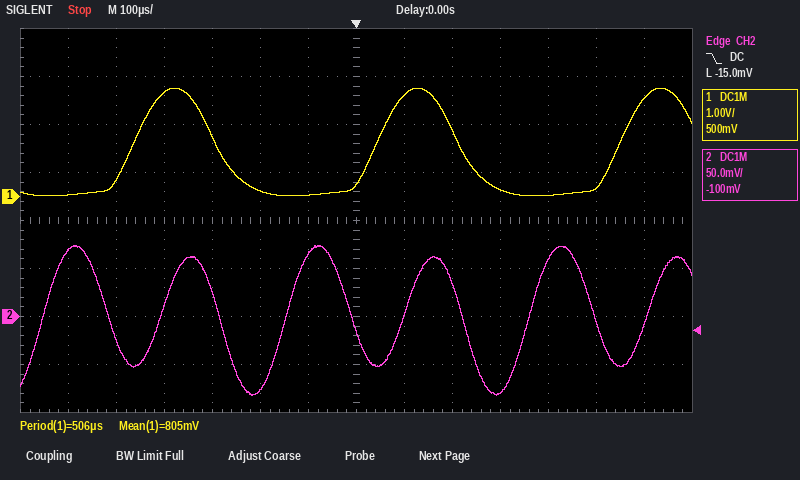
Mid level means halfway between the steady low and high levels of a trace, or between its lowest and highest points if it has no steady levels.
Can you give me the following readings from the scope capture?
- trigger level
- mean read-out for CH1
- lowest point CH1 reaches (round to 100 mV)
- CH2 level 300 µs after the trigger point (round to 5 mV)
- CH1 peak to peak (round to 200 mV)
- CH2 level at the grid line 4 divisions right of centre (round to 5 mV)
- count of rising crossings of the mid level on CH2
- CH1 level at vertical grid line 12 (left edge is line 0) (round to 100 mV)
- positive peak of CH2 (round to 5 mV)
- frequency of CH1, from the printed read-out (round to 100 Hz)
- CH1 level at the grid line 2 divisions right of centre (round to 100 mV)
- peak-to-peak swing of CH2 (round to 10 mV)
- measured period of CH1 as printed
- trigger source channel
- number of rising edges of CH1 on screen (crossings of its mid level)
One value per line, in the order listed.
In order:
-15.0 mV
805 mV
0.0 V
-80 mV
2.2 V
60 mV
6
200 mV
75 mV
2.0 kHz
1.4 V
160 mV
506 µs
CH2
3
